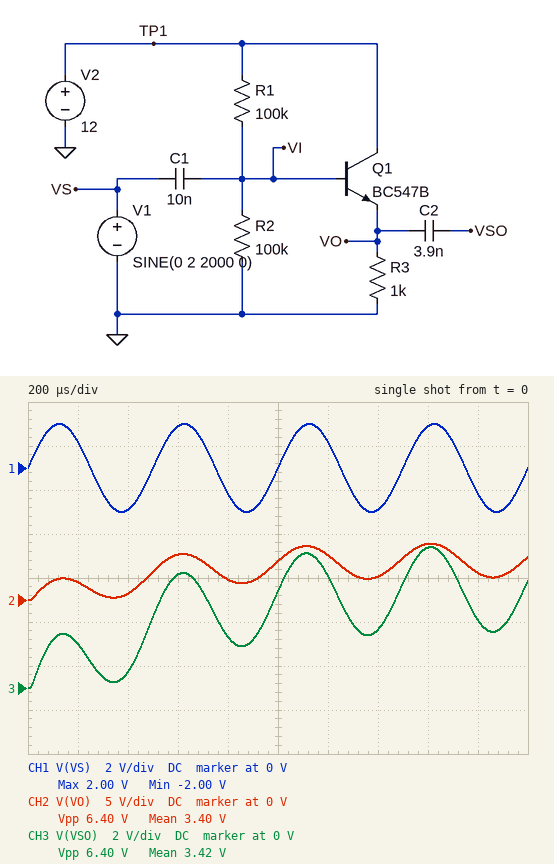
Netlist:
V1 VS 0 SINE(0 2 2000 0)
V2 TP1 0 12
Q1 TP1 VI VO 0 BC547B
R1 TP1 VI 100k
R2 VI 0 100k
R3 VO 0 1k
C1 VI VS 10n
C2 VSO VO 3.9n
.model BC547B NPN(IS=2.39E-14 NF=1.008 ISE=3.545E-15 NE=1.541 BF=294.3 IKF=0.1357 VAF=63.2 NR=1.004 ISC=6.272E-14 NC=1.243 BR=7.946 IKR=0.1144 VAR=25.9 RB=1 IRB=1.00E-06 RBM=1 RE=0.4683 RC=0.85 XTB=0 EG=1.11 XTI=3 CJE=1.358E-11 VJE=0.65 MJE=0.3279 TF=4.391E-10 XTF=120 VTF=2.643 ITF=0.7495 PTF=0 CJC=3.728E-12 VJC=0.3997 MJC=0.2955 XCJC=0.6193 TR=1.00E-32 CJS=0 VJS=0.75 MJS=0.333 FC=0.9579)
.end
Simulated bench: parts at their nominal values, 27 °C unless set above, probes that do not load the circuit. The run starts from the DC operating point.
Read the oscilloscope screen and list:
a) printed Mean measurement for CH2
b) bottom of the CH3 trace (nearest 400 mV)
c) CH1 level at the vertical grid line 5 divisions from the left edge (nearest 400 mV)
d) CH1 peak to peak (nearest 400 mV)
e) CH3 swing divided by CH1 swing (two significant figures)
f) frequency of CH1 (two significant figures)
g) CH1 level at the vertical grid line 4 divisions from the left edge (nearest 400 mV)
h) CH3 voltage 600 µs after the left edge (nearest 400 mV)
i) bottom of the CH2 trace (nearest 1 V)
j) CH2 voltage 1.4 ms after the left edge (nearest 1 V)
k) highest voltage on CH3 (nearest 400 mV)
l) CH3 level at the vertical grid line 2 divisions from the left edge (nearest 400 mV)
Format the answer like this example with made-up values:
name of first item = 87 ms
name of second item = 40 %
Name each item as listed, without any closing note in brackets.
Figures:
printed Mean measurement for CH2 = 3.40 V
bottom of the CH3 trace = 0 V
CH1 level at the vertical grid line 5 divisions from the left edge = 0 V
CH1 peak to peak = 4.0 V
CH3 swing divided by CH1 swing = 1.6
frequency of CH1 = 2.0 kHz
CH1 level at the vertical grid line 4 divisions from the left edge = -1.2 V
CH3 voltage 600 µs after the left edge = 5.2 V
bottom of the CH2 trace = 0 V
CH2 voltage 1.4 ms after the left edge = 3 V
highest voltage on CH3 = 6.4 V
CH3 level at the vertical grid line 2 divisions from the left edge = 800 mV
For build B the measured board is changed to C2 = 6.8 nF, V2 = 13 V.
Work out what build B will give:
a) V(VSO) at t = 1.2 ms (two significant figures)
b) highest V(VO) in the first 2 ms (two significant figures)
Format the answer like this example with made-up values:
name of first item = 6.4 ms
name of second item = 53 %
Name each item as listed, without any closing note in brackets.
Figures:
V(VSO) at t = 1.2 ms = 5.5 V
highest V(VO) in the first 2 ms = 6.8 V
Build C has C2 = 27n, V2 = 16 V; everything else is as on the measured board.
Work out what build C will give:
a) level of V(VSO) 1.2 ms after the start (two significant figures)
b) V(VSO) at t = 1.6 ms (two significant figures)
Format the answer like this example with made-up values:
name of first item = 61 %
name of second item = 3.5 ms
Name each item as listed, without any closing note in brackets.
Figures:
level of V(VSO) 1.2 ms after the start = 6.7 V
V(VSO) at t = 1.6 ms = 8.1 V
